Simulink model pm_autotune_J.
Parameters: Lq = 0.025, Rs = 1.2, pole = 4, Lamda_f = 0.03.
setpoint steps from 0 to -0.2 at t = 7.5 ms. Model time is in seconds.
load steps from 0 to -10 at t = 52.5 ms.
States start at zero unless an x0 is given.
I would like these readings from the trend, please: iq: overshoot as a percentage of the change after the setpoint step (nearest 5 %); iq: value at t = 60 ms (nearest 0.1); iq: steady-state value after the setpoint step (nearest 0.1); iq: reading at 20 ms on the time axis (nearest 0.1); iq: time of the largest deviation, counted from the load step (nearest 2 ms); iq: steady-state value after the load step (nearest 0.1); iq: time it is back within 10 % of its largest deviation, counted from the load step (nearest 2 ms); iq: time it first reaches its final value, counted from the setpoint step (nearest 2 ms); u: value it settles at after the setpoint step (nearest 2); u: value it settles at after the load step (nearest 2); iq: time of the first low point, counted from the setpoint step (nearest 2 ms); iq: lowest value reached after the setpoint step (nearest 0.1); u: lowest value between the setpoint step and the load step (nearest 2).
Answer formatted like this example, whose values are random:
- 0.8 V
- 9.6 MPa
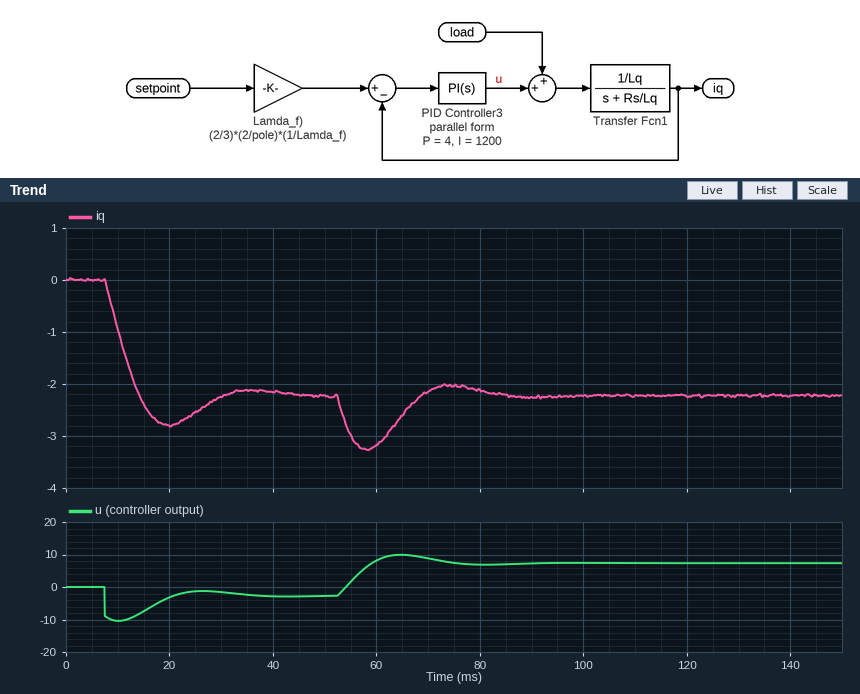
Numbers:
- 25 %
- -3.2
- -2.2
- -2.8
- 6 ms
- -2.2
- 28 ms
- 6 ms
- -2
- 8
- 12 ms
- -2.8
- -10
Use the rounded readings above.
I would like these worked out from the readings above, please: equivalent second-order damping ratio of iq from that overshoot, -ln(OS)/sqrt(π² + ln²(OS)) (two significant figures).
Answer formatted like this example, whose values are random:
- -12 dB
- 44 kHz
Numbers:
- 0.40
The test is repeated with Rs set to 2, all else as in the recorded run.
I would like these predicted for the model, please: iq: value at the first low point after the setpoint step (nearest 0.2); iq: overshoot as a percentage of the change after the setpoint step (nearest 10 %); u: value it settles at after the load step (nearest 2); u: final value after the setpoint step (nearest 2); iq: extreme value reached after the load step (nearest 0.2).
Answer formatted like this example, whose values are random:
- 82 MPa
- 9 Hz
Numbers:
- -2.6
- 20 %
- 6
- -4
- -3.2
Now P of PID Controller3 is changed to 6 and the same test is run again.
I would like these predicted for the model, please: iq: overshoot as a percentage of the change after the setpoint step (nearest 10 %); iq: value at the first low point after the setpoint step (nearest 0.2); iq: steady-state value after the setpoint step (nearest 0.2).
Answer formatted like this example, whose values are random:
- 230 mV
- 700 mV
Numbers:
- 20 %
- -2.6
- -2.2
